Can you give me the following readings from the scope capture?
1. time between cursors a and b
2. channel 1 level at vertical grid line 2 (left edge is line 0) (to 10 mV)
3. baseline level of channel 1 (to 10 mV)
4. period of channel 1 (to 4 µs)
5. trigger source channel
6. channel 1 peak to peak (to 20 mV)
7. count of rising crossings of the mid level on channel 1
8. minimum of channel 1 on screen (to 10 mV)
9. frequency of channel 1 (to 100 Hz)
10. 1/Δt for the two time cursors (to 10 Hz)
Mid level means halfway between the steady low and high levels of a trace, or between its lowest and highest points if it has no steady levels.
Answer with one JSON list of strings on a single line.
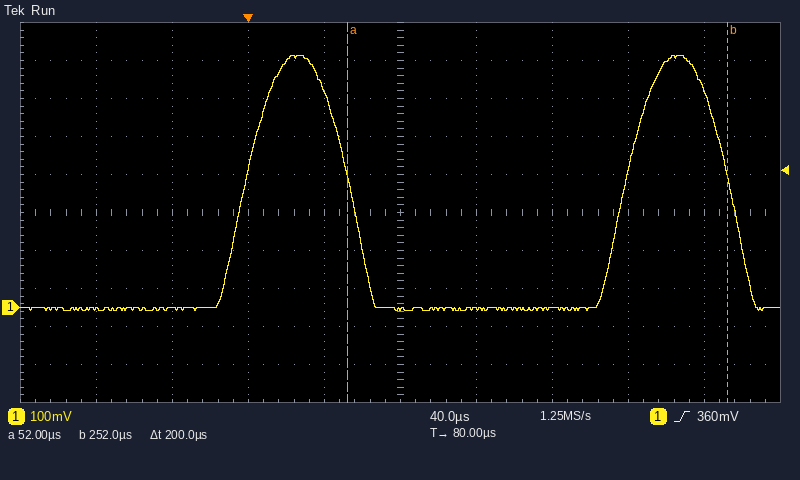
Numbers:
["200 µs", "0 mV", "0 mV", "200 µs", "channel 1", "680 mV", "2", "-10 mV", "5.0 kHz", "5.00 kHz"]
